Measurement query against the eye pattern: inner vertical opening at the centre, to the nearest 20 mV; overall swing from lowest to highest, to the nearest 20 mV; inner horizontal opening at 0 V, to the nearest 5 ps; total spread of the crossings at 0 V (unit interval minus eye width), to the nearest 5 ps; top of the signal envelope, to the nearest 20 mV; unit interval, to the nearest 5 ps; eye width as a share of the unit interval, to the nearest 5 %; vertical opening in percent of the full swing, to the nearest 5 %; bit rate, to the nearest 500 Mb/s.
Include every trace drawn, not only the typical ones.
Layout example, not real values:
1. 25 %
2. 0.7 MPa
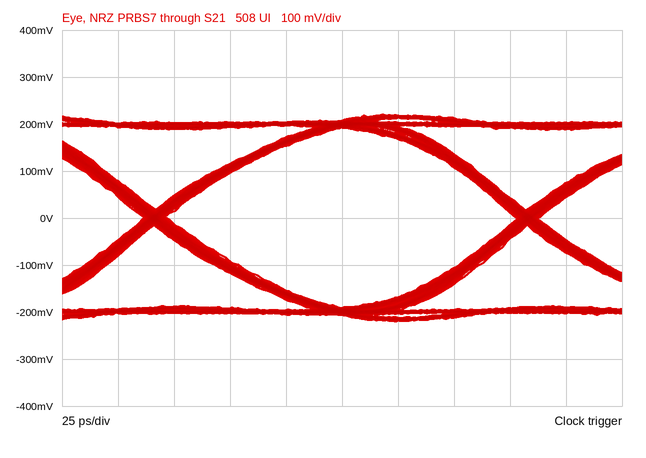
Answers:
1. 380 mV
2. 440 mV
3. 155 ps
4. 10 ps
5. 220 mV
6. 165 ps
7. 95 %
8. 85 %
9. 6.0 Gb/s
